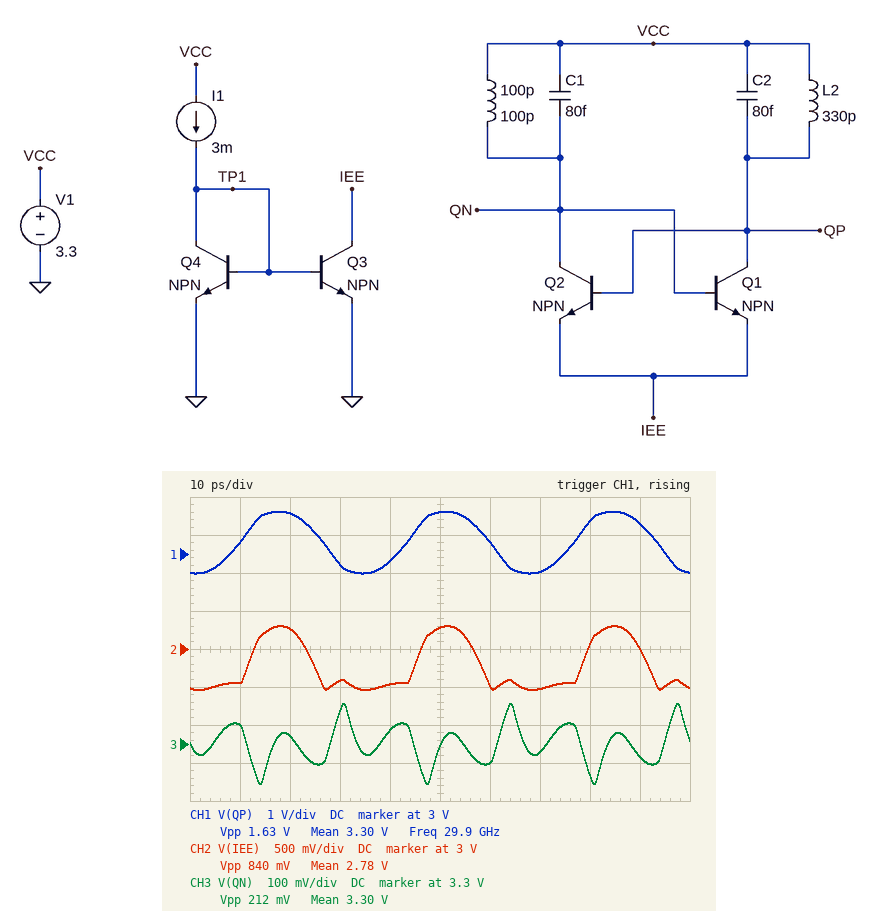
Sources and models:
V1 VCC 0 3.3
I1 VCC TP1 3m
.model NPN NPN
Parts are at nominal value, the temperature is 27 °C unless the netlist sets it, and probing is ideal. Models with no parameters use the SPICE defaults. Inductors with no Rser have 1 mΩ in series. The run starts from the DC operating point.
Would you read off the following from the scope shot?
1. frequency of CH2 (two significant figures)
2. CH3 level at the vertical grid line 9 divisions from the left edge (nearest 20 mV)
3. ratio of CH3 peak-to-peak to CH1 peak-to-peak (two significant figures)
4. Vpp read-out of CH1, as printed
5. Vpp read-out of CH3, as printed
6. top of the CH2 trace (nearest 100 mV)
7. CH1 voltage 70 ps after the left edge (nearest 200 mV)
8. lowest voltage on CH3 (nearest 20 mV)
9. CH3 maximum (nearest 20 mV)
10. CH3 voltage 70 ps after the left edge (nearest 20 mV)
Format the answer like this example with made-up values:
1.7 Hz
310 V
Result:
30 GHz
3.26 V
0.13
1.63 V
212 mV
3.3 V
2.6 V
3.20 V
3.40 V
3.28 V
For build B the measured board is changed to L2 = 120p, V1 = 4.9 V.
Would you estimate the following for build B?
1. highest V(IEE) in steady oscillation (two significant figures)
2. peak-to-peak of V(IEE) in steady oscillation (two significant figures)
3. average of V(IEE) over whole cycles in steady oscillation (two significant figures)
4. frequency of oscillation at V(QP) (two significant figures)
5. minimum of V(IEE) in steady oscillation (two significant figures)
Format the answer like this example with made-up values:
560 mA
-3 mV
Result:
5.1 V
1.2 V
4.4 V
55 GHz
3.9 V
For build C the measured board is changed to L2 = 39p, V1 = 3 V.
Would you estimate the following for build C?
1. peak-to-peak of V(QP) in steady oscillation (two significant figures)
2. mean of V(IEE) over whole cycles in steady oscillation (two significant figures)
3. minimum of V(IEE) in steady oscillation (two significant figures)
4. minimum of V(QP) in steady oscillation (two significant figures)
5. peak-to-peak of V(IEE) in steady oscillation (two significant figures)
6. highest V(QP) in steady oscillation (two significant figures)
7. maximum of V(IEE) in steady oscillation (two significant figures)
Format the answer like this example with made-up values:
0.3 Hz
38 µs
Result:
110 mV
2.5 V
2.2 V
2.9 V
820 mV
3.1 V
3.0 V
